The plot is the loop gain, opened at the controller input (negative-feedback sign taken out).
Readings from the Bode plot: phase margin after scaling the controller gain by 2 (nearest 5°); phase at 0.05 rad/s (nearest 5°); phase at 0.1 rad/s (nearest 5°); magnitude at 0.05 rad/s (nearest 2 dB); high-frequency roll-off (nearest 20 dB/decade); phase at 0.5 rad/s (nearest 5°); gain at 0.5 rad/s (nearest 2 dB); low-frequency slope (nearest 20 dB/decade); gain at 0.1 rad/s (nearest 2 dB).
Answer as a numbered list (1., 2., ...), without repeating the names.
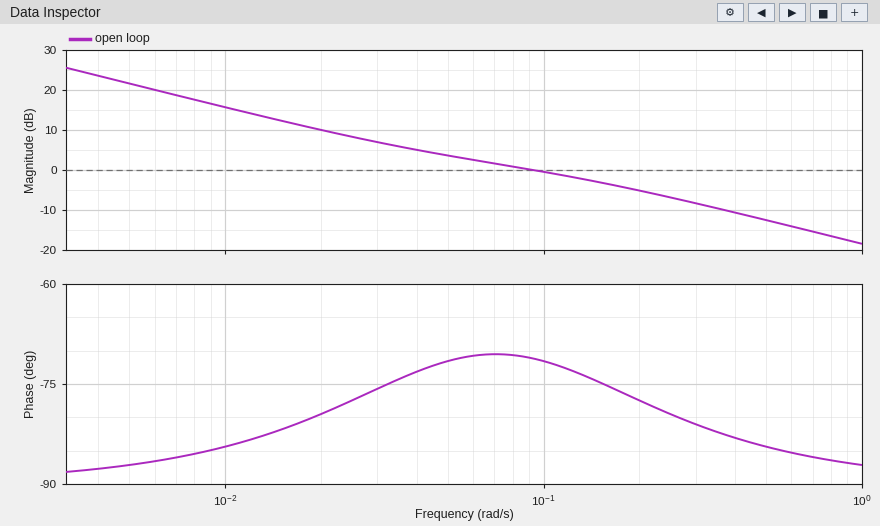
1. 100°
2. -70°
3. -70°
4. 4 dB
5. -20 dB/decade
6. -85°
7. -12 dB
8. -20 dB/decade
9. 0 dB
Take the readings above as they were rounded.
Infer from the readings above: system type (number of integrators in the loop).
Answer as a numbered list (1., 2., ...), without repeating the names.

1. 1
